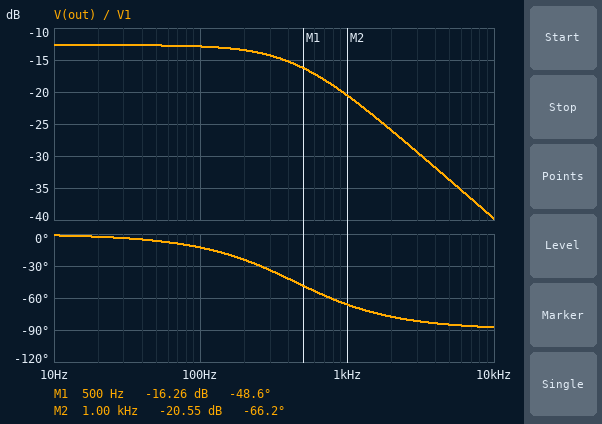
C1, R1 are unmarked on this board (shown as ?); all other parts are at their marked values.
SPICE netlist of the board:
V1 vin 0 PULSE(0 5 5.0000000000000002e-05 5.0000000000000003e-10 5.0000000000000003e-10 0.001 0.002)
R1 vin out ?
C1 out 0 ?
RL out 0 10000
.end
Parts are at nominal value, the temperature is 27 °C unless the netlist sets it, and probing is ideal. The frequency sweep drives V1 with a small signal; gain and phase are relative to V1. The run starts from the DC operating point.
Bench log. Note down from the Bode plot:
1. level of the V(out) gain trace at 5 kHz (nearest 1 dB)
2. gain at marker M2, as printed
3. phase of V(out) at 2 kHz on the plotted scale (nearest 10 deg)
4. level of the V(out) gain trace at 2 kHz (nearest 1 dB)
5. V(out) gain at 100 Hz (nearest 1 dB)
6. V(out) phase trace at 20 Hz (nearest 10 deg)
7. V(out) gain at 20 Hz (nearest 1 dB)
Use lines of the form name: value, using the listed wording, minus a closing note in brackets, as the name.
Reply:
level of the V(out) gain trace at 5 kHz: -34 dB
gain at marker M2, as printed: -20.55 dB
phase of V(out) at 2 kHz on the plotted scale: -80 deg
level of the V(out) gain trace at 2 kHz: -26 dB
V(out) gain at 100 Hz: -13 dB
V(out) phase trace at 20 Hz: 0 deg
V(out) gain at 20 Hz: -13 dB
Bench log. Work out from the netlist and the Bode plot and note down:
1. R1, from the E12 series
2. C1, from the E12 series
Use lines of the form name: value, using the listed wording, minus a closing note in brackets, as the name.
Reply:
R1, from the E12 series: 33 kΩ
C1, from the E12 series: 47 nF
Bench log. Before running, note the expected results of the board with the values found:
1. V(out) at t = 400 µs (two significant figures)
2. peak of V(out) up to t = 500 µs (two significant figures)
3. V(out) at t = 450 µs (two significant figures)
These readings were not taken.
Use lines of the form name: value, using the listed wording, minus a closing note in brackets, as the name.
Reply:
V(out) at t = 400 µs: 720 mV
peak of V(out) up to t = 500 µs: 830 mV
V(out) at t = 450 µs: 780 mV
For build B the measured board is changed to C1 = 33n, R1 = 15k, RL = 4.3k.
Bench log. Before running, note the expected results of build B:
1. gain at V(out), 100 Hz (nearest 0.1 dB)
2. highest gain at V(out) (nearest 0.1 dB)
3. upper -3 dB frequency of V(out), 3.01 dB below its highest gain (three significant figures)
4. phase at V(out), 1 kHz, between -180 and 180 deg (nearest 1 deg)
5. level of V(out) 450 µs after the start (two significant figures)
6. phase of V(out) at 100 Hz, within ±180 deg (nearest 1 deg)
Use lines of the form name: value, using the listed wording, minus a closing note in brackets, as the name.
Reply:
gain at V(out), 100 Hz: -13.1 dB
highest gain at V(out): -13.0 dB
upper -3 dB frequency of V(out), 3.01 dB below its highest gain: 1.44 kHz
phase at V(out), 1 kHz, between -180 and 180 deg: -35 deg
level of V(out) 450 µs after the start: 1.1 V
phase of V(out) at 100 Hz, within ±180 deg: -4 deg
